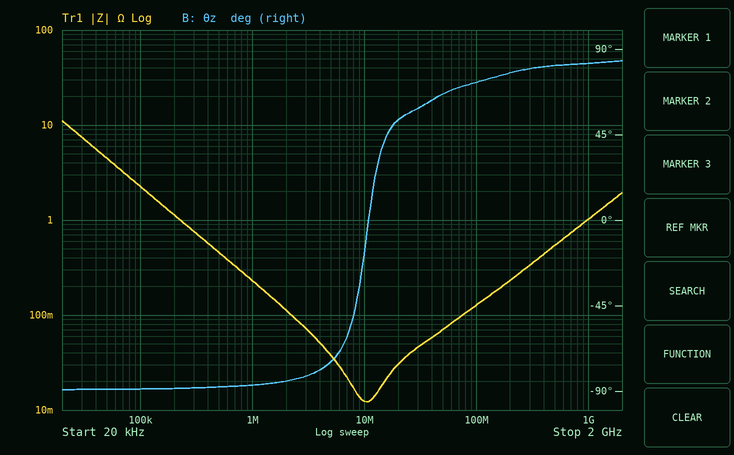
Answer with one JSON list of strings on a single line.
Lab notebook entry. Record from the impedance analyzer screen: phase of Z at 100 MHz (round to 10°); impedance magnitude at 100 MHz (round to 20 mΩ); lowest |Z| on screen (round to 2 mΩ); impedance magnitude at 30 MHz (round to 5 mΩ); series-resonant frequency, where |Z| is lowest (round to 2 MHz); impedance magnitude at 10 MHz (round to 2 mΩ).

["70°", "120 mΩ", "12 mΩ", "45 mΩ", "10 MHz", "12 mΩ"]
